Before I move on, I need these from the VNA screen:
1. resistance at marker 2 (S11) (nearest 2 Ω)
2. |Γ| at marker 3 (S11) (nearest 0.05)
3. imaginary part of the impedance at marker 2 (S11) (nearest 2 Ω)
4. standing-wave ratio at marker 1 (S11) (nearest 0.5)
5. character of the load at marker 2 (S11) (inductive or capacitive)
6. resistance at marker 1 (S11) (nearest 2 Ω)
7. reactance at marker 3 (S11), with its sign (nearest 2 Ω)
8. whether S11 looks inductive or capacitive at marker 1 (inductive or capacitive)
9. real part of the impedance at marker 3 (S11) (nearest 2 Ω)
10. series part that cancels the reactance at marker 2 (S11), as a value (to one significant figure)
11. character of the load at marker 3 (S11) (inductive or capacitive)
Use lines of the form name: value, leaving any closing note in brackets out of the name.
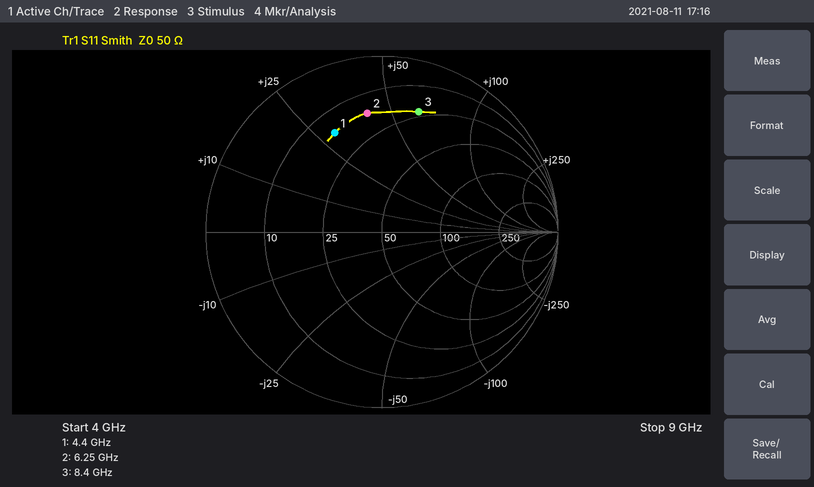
resistance at marker 2 (S11): 16 Ω
|Γ| at marker 3 (S11): 0.70
imaginary part of the impedance at marker 2 (S11): +42 Ω
standing-wave ratio at marker 1 (S11): 4.5
character of the load at marker 2 (S11): inductive
resistance at marker 1 (S11): 16 Ω
reactance at marker 3 (S11), with its sign: +62 Ω
whether S11 looks inductive or capacitive at marker 1: inductive
real part of the impedance at marker 3 (S11): 22 Ω
series part that cancels the reactance at marker 2 (S11), as a value: 600 fF
character of the load at marker 3 (S11): inductive
